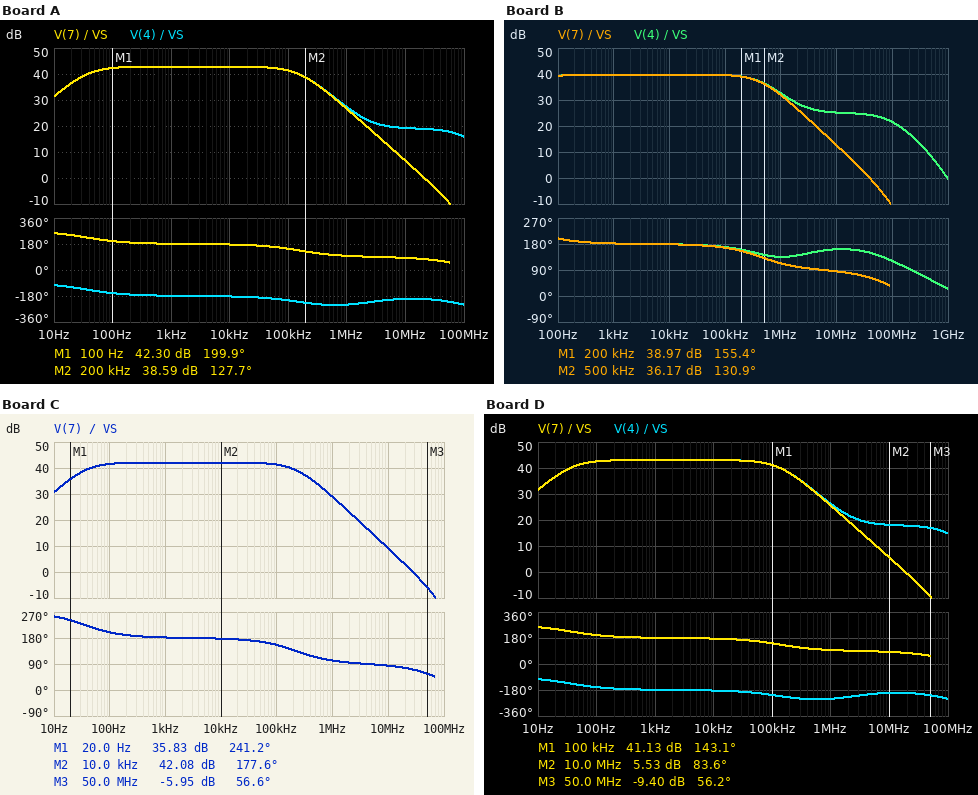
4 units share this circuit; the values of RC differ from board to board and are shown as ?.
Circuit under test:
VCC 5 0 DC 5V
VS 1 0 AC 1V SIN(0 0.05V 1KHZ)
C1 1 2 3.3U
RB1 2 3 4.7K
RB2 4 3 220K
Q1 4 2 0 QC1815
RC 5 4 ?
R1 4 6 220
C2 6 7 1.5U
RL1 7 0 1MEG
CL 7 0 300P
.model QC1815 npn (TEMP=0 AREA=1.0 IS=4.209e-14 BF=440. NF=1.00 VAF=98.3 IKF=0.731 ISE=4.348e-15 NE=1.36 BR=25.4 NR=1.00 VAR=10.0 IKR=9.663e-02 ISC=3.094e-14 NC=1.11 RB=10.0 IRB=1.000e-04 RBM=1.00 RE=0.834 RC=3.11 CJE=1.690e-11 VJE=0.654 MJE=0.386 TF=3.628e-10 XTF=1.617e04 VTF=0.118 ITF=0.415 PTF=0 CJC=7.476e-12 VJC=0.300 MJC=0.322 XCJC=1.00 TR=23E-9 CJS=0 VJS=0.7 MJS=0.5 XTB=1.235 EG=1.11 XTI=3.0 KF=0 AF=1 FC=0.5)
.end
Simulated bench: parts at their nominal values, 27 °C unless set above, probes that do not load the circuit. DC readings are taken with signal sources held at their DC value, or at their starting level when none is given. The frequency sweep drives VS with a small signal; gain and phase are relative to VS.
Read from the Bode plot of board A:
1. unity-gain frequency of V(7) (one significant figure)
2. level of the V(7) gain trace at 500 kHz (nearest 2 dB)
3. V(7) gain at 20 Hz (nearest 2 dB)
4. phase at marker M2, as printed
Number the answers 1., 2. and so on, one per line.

1. 20 MHz
2. 32 dB
3. 36 dB
4. 127.7 deg
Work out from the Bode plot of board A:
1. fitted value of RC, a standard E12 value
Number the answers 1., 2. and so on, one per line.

1. 3.3 kΩ
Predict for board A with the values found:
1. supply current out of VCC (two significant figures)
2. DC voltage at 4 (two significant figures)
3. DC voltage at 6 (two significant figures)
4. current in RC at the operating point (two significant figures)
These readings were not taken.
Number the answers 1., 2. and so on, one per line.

1. 1.1 mA
2. 1.4 V
3. 1.4 V
4. 1.1 mA
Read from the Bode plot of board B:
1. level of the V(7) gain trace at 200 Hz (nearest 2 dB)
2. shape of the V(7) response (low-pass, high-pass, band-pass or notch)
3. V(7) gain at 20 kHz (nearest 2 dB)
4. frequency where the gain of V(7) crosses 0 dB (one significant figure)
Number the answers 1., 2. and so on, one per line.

1. 40 dB
2. low-pass
3. 40 dB
4. 40 MHz
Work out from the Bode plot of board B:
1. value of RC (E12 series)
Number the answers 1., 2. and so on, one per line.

1. 1 kΩ
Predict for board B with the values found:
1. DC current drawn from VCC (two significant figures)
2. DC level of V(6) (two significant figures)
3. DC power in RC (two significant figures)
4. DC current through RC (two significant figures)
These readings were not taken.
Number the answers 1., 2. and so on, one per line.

1. 2.6 mA
2. 2.4 V
3. 6.9 mW
4. 2.6 mA
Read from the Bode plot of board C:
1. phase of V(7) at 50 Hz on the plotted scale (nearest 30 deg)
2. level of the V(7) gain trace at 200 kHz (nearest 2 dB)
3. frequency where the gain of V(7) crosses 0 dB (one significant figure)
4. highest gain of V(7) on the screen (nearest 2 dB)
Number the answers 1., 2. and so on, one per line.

1. 210 deg
2. 40 dB
3. 30 MHz
4. 42 dB
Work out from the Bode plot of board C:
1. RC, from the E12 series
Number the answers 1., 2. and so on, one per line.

1. 2.2 kΩ
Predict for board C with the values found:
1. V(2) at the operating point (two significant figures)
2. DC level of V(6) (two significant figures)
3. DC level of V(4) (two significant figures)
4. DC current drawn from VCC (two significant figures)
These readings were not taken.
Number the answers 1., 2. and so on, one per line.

1. 680 mV
2. 1.7 V
3. 1.7 V
4. 1.5 mA
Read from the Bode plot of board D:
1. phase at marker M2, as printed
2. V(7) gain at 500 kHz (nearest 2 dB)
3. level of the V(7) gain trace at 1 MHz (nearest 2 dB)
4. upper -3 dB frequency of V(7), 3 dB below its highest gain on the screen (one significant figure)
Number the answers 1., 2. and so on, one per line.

1. 83.6 deg
2. 32 dB
3. 26 dB
4. 100 kHz
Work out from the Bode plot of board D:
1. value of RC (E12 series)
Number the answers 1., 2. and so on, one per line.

1. 3.9 kΩ
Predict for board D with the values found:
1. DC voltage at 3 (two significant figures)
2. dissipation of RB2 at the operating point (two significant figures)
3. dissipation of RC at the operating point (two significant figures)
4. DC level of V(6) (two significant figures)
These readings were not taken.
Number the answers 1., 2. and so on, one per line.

1. 680 mV
2. 1.7 µW
3. 3.5 mW
4. 1.3 V
